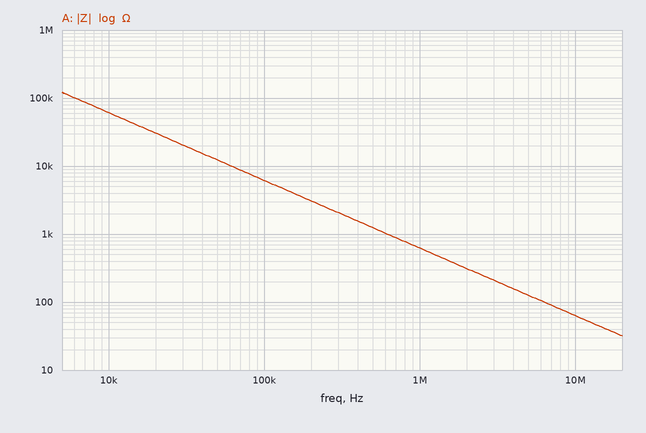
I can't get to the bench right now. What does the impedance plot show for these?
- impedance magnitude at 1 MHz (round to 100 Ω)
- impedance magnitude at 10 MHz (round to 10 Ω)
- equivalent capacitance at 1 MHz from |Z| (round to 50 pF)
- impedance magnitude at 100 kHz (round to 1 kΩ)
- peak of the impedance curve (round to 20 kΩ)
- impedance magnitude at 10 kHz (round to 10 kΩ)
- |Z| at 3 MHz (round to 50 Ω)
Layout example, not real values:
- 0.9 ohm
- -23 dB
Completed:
- 600 Ω
- 60 Ω
- 250 pF
- 6 kΩ
- 120 kΩ
- 60 kΩ
- 200 Ω
